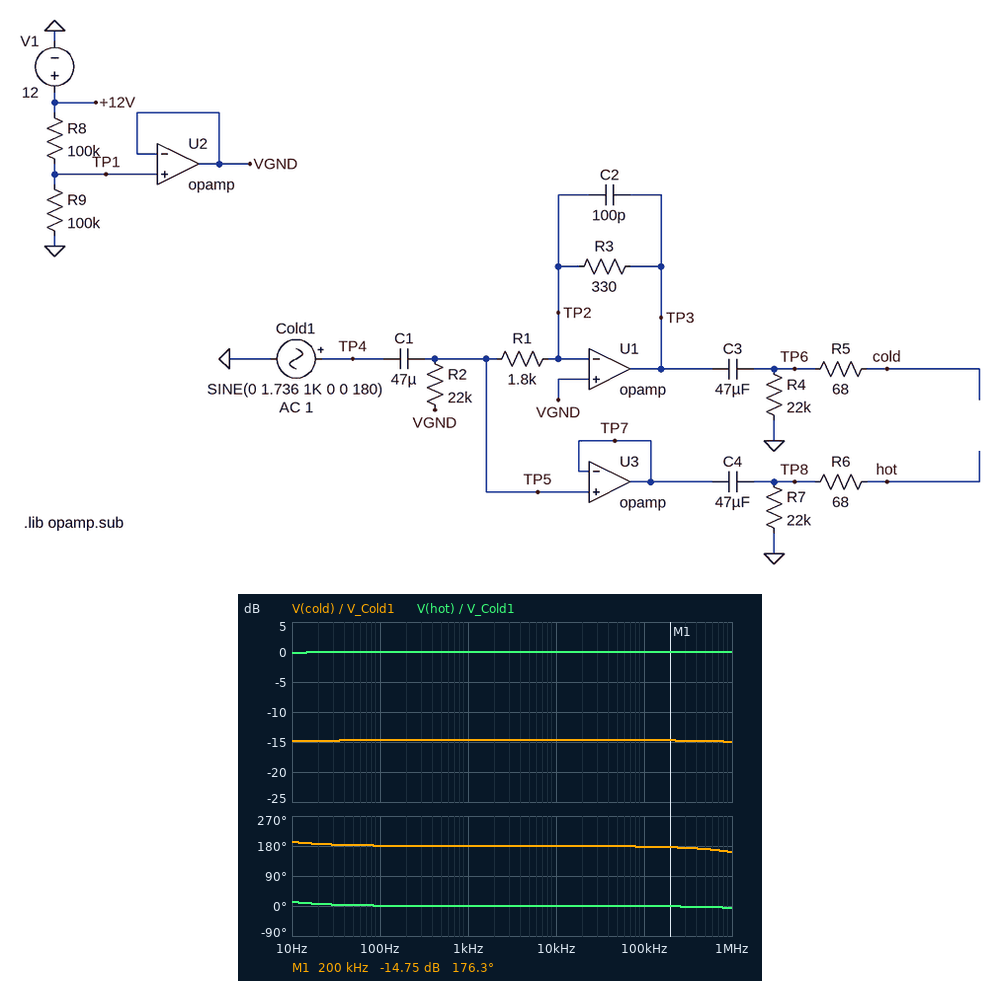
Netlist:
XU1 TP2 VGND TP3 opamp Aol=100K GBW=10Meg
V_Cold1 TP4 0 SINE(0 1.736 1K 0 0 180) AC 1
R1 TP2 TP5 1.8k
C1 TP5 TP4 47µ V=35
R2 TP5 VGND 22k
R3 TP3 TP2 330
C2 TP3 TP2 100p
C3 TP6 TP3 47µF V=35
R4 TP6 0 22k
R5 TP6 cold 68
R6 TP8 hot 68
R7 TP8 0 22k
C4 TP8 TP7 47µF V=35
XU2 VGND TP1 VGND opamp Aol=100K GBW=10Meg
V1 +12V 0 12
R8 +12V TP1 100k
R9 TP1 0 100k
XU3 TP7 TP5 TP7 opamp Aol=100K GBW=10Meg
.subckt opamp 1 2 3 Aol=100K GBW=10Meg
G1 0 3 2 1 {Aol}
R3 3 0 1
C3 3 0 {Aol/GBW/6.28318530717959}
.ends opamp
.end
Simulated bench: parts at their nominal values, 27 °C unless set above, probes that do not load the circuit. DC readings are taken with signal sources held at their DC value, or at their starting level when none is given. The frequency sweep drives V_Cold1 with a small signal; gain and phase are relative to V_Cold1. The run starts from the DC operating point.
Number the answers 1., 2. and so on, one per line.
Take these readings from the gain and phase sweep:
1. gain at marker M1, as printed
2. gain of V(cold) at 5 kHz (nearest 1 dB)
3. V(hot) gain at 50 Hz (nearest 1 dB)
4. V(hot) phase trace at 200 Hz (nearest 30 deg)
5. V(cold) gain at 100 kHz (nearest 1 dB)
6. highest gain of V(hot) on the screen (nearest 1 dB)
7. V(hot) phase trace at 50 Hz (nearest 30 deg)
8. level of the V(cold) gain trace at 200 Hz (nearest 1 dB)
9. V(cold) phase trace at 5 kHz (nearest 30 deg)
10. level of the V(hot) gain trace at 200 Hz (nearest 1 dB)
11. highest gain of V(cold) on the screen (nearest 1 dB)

1. -14.75 dB
2. -15 dB
3. 0 dB
4. 0 deg
5. -15 dB
6. 0 dB
7. 0 deg
8. -15 dB
9. 180 deg
10. 0 dB
11. -15 dB
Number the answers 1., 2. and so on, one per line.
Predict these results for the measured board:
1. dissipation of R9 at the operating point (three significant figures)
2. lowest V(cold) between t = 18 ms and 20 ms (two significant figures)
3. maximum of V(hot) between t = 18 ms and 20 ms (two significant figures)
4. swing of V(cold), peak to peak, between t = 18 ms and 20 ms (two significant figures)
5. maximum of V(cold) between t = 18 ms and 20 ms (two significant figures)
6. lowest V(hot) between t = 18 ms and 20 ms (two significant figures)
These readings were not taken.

1. 360 µW
2. -320 mV
3. 1.7 V
4. 640 mV
5. 320 mV
6. -1.7 V
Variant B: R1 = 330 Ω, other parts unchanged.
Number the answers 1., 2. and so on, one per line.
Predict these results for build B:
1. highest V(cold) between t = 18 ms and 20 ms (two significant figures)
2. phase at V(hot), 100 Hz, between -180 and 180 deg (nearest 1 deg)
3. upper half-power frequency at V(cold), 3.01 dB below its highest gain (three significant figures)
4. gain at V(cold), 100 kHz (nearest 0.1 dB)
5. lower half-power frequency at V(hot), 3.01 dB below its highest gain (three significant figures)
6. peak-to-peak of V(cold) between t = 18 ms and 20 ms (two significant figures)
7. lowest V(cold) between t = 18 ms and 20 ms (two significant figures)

1. 1.7 V
2. 6 deg
3. 2.80 MHz
4. 0 dB
5. 10.4 Hz
6. 3.5 V
7. -1.7 V
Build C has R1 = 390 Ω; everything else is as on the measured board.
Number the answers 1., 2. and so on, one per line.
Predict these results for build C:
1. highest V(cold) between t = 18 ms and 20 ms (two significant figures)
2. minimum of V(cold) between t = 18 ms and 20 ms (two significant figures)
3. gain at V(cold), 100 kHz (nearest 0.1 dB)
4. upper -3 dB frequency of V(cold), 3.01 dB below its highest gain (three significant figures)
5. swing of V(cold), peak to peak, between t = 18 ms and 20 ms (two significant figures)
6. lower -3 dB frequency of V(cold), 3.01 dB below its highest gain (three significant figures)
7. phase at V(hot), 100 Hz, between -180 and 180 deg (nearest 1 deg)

1. 1.5 V
2. -1.5 V
3. -1.5 dB
4. 2.94 MHz
5. 2.9 V
6. 8.84 Hz
7. 5 deg
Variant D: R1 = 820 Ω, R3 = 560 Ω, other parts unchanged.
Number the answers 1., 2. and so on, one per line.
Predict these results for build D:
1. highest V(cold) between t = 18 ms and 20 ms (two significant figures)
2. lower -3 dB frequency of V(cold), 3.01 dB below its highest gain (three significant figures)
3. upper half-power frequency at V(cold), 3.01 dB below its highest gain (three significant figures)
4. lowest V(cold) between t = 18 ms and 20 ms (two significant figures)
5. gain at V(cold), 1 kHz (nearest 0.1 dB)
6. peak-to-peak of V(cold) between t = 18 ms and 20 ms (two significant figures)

1. 1.2 V
2. 4.29 Hz
3. 2.20 MHz
4. -1.2 V
5. -3.3 dB
6. 2.4 V
